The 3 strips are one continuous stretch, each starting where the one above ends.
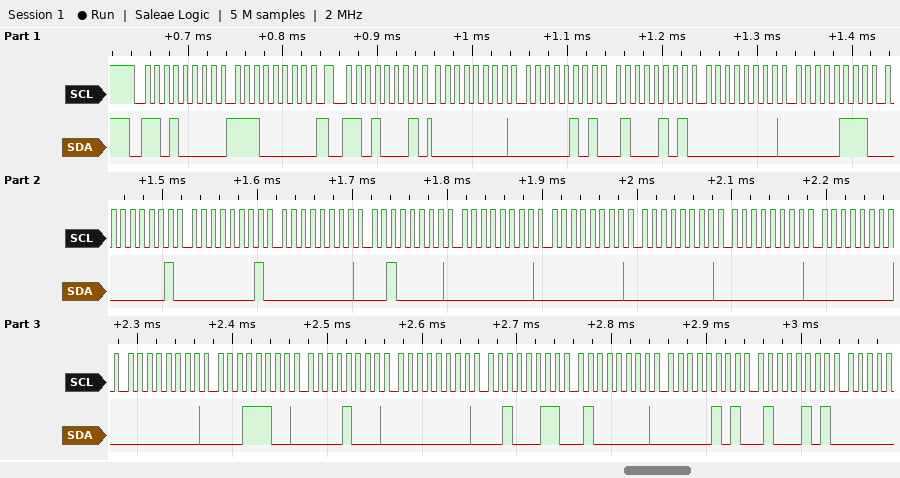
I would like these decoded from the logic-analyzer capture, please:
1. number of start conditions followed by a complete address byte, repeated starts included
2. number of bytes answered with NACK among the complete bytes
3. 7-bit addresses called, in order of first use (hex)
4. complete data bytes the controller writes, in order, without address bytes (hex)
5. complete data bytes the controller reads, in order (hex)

2
0
0x68
E0
00 05 45 00 07 01 01 00 20 00 00 00 00 00 00 1C 08 00 23 40 05 45
